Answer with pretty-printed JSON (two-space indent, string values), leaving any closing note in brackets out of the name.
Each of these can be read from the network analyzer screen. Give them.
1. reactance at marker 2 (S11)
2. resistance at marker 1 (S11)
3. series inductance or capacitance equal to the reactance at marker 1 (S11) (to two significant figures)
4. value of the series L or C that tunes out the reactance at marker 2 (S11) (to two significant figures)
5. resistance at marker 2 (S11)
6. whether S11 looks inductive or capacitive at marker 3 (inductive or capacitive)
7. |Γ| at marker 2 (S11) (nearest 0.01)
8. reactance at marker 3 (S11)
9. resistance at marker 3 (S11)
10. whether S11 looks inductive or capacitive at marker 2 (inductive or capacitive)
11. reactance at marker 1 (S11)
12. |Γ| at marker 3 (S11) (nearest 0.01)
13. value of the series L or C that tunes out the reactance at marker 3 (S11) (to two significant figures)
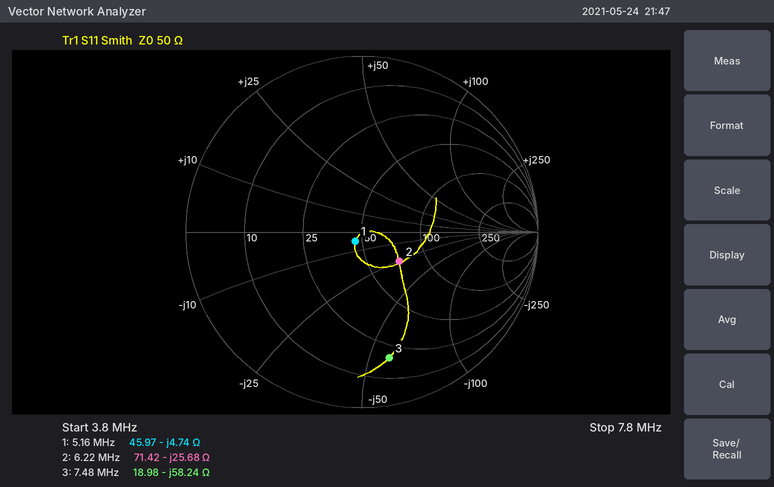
{
  "reactance at marker 2": "-25.68 Ω",
  "resistance at marker 1": "45.97 Ω",
  "series inductance or capacitance equal to the reactance at marker 1 (S11)": "6.5 nF",
  "value of the series L or C that tunes out the reactance at marker 2 (S11)": "660 nH",
  "resistance at marker 2": "71.42 Ω",
  "whether S11 looks inductive or capacitive at marker 3": "capacitive",
  "|Γ| at marker 2 (S11)": "0.27",
  "reactance at marker 3": "-58.24 Ω",
  "resistance at marker 3": "18.98 Ω",
  "whether S11 looks inductive or capacitive at marker 2": "capacitive",
  "reactance at marker 1": "-4.74 Ω",
  "|Γ| at marker 3 (S11)": "0.73",
  "value of the series L or C that tunes out the reactance at marker 3 (S11)": "1.2 µH"
}
